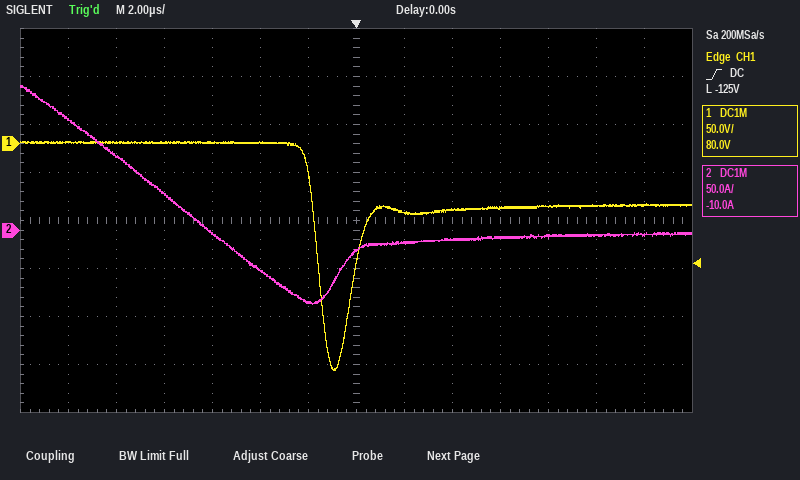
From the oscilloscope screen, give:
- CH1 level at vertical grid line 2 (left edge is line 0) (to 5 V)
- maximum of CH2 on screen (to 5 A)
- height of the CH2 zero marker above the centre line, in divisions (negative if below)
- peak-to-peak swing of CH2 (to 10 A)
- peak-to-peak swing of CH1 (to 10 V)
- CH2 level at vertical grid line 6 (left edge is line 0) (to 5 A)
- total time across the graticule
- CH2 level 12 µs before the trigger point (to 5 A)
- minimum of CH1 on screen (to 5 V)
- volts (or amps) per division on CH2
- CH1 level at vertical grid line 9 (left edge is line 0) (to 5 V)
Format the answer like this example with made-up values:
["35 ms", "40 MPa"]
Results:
["0 V", "150 A", "-0.2 div", "230 A", "240 V", "-75 A", "28 µs", "115 A", "-235 V", "50 A", "-70 V"]
